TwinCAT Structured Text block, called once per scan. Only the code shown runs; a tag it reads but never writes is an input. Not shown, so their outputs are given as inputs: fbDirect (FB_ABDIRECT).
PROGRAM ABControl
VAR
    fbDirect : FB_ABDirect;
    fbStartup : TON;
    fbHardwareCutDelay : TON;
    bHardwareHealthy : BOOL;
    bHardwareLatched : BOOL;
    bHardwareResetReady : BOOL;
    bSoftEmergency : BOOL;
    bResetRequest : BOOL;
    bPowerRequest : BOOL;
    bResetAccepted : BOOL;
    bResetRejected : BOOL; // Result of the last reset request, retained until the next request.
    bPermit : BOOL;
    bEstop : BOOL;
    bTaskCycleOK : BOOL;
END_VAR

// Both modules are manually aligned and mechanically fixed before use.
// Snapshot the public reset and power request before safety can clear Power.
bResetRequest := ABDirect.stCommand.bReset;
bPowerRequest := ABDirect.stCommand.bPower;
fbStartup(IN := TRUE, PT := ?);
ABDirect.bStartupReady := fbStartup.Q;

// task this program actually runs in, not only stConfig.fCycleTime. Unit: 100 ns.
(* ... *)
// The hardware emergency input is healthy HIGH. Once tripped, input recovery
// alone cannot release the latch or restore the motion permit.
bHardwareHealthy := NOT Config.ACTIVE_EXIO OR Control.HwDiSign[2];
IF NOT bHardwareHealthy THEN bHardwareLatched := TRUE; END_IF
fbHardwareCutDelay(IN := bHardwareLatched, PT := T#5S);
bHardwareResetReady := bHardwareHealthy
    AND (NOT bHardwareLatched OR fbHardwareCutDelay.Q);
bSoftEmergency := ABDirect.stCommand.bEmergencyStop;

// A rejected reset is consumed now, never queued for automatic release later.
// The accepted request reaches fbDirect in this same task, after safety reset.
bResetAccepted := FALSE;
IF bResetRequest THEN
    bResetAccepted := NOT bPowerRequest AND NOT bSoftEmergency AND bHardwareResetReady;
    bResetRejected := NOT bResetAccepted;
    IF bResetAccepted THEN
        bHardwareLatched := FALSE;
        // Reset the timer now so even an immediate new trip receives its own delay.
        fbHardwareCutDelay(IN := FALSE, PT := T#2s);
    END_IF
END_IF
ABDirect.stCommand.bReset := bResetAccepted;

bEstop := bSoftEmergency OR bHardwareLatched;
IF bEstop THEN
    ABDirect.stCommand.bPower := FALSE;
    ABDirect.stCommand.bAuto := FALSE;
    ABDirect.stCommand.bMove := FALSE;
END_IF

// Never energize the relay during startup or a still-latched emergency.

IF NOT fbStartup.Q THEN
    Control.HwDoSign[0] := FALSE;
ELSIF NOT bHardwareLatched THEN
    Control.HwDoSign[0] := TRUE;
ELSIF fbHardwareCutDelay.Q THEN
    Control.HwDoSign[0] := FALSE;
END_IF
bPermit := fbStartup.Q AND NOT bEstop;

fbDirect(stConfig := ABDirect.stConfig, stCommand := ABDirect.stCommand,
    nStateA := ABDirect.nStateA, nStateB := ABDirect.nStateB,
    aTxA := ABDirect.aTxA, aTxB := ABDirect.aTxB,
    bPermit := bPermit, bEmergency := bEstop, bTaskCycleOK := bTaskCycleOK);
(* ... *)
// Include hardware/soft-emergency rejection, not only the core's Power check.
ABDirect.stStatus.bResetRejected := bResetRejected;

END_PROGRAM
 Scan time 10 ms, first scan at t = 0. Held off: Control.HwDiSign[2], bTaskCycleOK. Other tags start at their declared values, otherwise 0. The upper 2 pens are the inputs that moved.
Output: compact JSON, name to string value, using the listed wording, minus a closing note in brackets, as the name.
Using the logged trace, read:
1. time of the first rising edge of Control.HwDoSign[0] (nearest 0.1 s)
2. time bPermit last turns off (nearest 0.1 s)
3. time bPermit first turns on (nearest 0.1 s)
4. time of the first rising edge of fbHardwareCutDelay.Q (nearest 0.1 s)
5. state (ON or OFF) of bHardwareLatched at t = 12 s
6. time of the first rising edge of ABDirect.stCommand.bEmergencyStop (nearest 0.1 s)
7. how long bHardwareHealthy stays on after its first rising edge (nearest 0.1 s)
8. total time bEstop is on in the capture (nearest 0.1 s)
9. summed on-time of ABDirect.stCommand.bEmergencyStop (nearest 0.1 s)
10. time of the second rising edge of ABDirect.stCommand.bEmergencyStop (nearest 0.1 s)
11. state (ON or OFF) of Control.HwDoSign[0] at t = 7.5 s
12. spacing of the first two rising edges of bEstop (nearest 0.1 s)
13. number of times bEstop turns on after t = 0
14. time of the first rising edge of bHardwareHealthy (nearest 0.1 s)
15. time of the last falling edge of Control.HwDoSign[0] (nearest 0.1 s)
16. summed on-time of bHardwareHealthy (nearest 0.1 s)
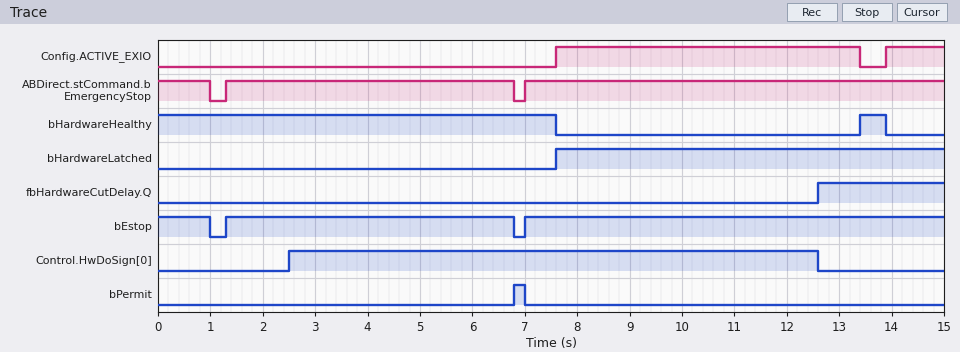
{"time of the first rising edge of Control.HwDoSign[0]": "2.5 s", "time bPermit last turns off": "7.0 s", "time bPermit first turns on": "6.8 s", "time of the first rising edge of fbHardwareCutDelay.Q": "12.6 s", "state (ON or OFF) of bHardwareLatched at t = 12 s": "ON", "time of the first rising edge of ABDirect.stCommand.bEmergencyStop": "1.3 s", "how long bHardwareHealthy stays on after its first rising edge": "0.5 s", "total time bEstop is on in the capture": "14.5 s", "summed on-time of ABDirect.stCommand.bEmergencyStop": "14.5 s", "time of the second rising edge of ABDirect.stCommand.bEmergencyStop": "7.0 s", "state (ON or OFF) of Control.HwDoSign[0] at t = 7.5 s": "ON", "spacing of the first two rising edges of bEstop": "5.7 s", "number of times bEstop turns on after t = 0": "2", "time of the first rising edge of bHardwareHealthy": "13.4 s", "time of the last falling edge of Control.HwDoSign[0]": "12.6 s", "summed on-time of bHardwareHealthy": "8.1 s"}
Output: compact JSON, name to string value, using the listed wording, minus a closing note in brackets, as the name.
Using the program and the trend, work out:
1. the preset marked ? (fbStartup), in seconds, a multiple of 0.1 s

{"the preset marked ? (fbStartup), in seconds, a multiple of 0.1 s": "2.5 s"}
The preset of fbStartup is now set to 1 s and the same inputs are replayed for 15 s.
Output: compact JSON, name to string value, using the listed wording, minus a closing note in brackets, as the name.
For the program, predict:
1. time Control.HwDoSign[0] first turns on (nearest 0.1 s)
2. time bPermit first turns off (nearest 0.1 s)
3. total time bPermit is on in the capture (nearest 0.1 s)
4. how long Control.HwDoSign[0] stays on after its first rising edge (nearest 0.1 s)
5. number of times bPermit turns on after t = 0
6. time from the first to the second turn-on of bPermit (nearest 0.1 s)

{"time Control.HwDoSign[0] first turns on": "1.0 s", "time bPermit first turns off": "1.3 s", "total time bPermit is on in the capture": "0.5 s", "how long Control.HwDoSign[0] stays on after its first rising edge": "11.6 s", "number of times bPermit turns on after t = 0": "2", "time from the first to the second turn-on of bPermit": "5.8 s"}
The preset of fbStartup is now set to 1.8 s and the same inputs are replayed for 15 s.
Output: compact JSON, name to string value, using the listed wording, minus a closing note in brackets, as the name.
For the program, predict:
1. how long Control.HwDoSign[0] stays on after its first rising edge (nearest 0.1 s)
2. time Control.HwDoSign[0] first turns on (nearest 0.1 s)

{"how long Control.HwDoSign[0] stays on after its first rising edge": "10.8 s", "time Control.HwDoSign[0] first turns on": "1.8 s"}
